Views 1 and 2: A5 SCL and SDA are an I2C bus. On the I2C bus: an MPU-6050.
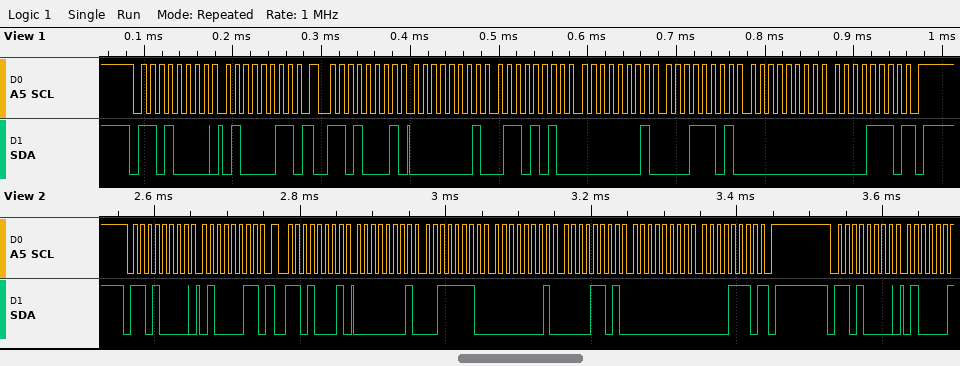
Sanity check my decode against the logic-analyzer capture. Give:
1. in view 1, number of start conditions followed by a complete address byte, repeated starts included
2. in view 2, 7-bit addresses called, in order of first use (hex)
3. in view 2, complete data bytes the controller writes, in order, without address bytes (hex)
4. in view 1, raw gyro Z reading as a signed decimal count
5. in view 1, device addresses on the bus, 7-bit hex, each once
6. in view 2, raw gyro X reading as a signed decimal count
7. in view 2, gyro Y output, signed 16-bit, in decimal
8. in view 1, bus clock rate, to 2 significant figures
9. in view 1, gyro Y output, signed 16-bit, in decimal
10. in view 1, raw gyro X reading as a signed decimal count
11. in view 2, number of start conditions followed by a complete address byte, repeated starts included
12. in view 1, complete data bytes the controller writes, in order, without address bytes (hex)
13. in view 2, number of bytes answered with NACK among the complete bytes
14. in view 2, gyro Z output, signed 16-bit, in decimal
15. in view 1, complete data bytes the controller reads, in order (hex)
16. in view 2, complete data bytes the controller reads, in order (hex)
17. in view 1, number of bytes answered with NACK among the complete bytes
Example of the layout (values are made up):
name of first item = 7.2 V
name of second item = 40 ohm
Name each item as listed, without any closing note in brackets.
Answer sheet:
in view 1, number of start conditions followed by a complete address byte, repeated starts included = 2
in view 2, 7-bit addresses called, in order of first use = 0x68
in view 2, complete data bytes the controller writes, in order, without address bytes = 43
in view 1, raw gyro Z reading as a signed decimal count = 14
in view 1, device addresses on the bus, 7-bit hex, each once = 0x68
in view 2, raw gyro X reading as a signed decimal count = 318
in view 2, gyro Y output, signed 16-bit, in decimal = 269
in view 1, bus clock rate, to 2 significant figures = 100 kHz
in view 1, gyro Y output, signed 16-bit, in decimal = 285
in view 1, raw gyro X reading as a signed decimal count = 362
in view 2, number of start conditions followed by a complete address byte, repeated starts included = 3
in view 1, complete data bytes the controller writes, in order, without address bytes = 43
in view 2, number of bytes answered with NACK among the complete bytes = 1
in view 2, gyro Z output, signed 16-bit, in decimal = 14
in view 1, complete data bytes the controller reads, in order = 01 6A 01 1D 00 0E
in view 2, complete data bytes the controller reads, in order = 01 3E 01 0D 00 0E
in view 1, number of bytes answered with NACK among the complete bytes = 1
